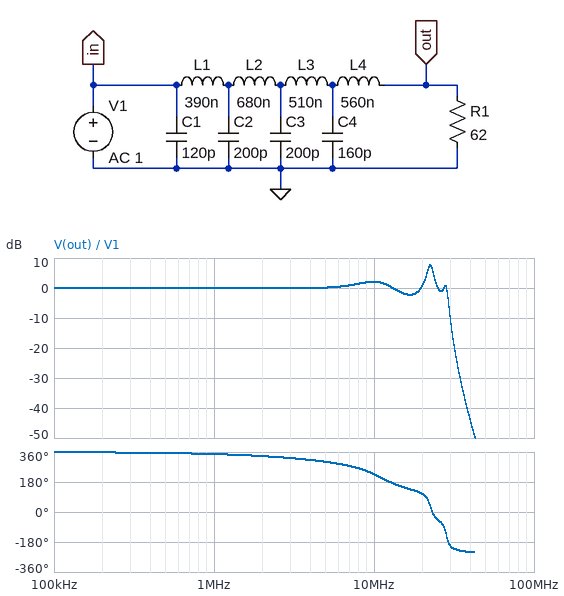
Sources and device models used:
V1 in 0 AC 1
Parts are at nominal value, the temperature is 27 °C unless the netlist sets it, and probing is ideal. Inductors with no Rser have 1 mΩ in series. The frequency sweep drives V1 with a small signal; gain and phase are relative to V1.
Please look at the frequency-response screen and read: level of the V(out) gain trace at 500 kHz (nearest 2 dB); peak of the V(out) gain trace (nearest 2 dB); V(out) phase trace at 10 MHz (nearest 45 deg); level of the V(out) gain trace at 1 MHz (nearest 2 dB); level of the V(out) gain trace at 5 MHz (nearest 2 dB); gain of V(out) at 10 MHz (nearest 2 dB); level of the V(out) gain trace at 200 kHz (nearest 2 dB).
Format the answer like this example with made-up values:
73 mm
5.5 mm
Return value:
0 dB
8 dB
225 deg
0 dB
0 dB
2 dB
0 dB
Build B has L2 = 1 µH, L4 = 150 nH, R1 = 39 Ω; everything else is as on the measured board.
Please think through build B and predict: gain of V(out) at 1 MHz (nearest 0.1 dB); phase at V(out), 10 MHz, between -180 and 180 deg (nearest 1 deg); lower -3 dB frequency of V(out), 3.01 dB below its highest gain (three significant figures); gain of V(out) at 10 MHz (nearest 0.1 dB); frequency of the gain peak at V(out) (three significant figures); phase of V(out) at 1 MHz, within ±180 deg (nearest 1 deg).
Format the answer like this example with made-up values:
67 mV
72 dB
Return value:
-0.2 dB
-119 deg
20.8 MHz
-4.2 dB
22.4 MHz
-19 deg
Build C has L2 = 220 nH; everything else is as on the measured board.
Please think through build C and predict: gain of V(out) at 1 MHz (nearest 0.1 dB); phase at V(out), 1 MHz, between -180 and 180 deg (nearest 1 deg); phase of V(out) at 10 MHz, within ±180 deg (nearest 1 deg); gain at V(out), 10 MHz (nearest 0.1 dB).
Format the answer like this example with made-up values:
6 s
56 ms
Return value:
0 dB
-10 deg
-105 deg
4.2 dB
